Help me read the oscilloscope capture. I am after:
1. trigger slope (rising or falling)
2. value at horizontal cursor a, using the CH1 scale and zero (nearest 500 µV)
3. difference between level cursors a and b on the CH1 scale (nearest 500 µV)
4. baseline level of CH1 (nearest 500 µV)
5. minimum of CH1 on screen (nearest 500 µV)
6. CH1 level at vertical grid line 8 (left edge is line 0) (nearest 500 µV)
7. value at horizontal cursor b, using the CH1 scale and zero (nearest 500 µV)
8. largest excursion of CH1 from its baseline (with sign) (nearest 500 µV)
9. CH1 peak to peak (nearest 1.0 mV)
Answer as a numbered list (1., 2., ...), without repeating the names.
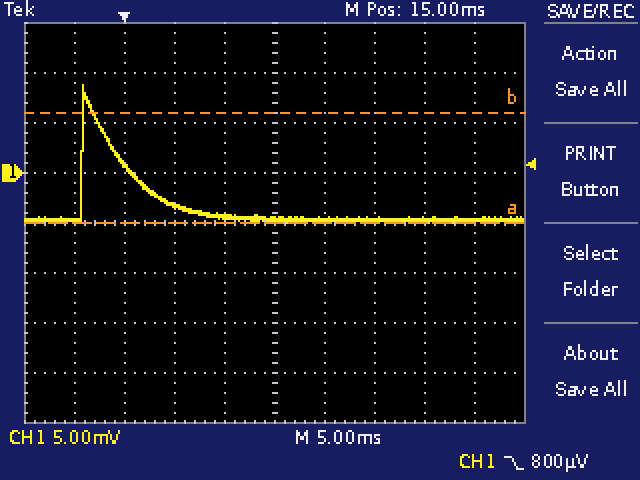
1. falling
2. -5.0 mV
3. 11.0 mV
4. -4.5 mV
5. -5.0 mV
6. -4.5 mV
7. 6.0 mV
8. +13.5 mV
9. 14.0 mV
